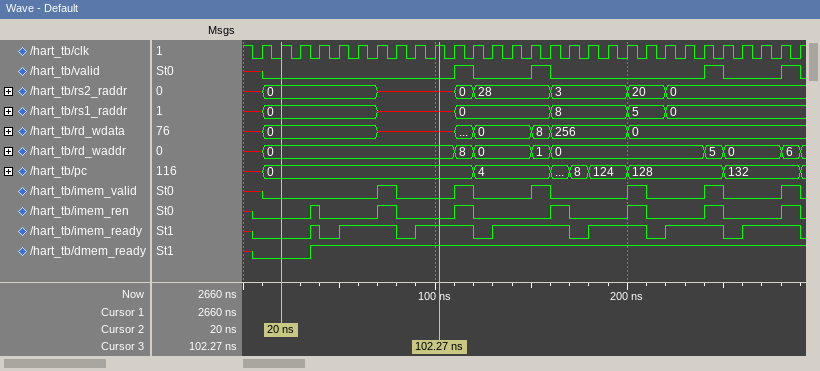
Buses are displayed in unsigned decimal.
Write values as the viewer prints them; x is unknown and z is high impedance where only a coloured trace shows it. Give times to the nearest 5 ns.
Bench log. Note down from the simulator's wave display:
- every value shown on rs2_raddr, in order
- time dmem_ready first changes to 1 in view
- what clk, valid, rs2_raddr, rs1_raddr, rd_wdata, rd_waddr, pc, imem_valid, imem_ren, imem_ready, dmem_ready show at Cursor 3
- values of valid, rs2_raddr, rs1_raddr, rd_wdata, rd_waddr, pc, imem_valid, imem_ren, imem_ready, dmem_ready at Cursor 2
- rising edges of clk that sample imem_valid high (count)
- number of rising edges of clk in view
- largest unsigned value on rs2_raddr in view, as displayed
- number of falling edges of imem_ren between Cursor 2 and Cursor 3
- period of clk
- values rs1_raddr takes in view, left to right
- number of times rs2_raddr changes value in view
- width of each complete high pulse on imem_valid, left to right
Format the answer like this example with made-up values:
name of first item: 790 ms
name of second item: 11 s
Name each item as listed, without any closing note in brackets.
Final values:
every value shown on rs2_raddr, in order: x, 0, x, 0, 28, 3, 20, 0
time dmem_ready first changes to 1 in view: 35 ns
what clk, valid, rs2_raddr, rs1_raddr, rd_wdata, rd_waddr, pc, imem_valid, imem_ren, imem_ready, dmem_ready show at Cursor 3: clk=1, valid=0, rs2_raddr=x, rs1_raddr=x, rd_wdata=x, rd_waddr=0, pc=0, imem_valid=0, imem_ren=0, imem_ready=1, dmem_ready=1
values of valid, rs2_raddr, rs1_raddr, rd_wdata, rd_waddr, pc, imem_valid, imem_ren, imem_ready, dmem_ready at Cursor 2: valid=0, rs2_raddr=0, rs1_raddr=0, rd_wdata=0, rd_waddr=0, pc=0, imem_valid=0, imem_ren=0, imem_ready=0, dmem_ready=0
rising edges of clk that sample imem_valid high: 6
number of rising edges of clk in view: 29
largest unsigned value on rs2_raddr in view, as displayed: 28
number of falling edges of imem_ren between Cursor 2 and Cursor 3: 2
period of clk: 10 ns
values rs1_raddr takes in view, left to right: x, 0, x, 0, 8, 5, 0
number of times rs2_raddr changes value in view: 7
width of each complete high pulse on imem_valid, left to right: 10 ns, 10 ns, 10 ns, 10 ns, 10 ns, 10 ns
